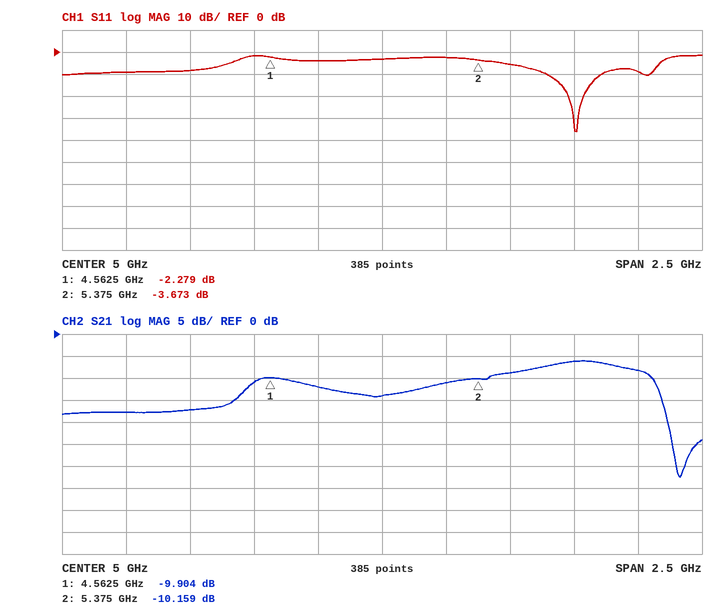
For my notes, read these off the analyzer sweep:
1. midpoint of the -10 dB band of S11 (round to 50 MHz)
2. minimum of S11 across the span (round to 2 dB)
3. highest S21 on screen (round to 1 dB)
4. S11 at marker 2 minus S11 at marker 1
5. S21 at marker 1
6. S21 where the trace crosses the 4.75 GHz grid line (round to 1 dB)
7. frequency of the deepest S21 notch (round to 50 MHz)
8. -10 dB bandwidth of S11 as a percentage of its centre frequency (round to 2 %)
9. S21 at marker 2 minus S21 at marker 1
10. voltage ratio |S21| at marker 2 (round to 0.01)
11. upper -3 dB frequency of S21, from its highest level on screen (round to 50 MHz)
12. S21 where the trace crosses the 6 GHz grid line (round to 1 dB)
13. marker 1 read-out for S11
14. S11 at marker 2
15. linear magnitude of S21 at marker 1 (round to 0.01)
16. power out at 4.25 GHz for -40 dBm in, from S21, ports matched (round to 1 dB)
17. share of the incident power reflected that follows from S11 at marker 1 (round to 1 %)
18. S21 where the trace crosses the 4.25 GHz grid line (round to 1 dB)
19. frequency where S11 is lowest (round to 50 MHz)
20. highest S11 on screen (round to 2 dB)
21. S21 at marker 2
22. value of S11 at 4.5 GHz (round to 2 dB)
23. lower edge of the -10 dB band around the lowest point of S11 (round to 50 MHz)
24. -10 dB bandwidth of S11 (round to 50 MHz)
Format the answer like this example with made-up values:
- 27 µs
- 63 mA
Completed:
- 5.75 GHz
- -36 dB
- -6 dB
- -1.394 dB
- -9.904 dB
- -12 dB
- 6.15 GHz
- 4 %
- -0.255 dB
- 0.31
- 6.05 GHz
- -8 dB
- -2.279 dB
- -3.673 dB
- 0.32
- -57 dBm
- 59 %
- -17 dB
- 5.75 GHz
- -2 dB
- -10.159 dB
- -2 dB
- 5.65 GHz
- 200 MHz
